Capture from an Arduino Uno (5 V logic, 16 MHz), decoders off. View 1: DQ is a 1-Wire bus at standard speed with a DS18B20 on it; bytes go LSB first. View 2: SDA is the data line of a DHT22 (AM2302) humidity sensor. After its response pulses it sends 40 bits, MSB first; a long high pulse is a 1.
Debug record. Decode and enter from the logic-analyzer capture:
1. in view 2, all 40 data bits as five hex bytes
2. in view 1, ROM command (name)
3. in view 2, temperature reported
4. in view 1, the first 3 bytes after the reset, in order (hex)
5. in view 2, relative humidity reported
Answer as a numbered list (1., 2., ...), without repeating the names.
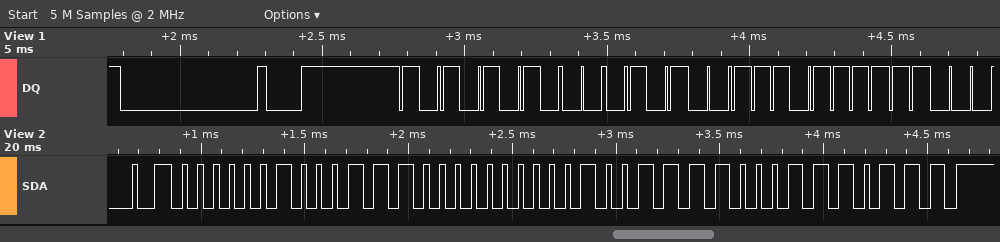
1. 02 38 01 3C 77
2. Match ROM
3. 31.6 °C
4. 55 28 F7
5. 56.8 %
